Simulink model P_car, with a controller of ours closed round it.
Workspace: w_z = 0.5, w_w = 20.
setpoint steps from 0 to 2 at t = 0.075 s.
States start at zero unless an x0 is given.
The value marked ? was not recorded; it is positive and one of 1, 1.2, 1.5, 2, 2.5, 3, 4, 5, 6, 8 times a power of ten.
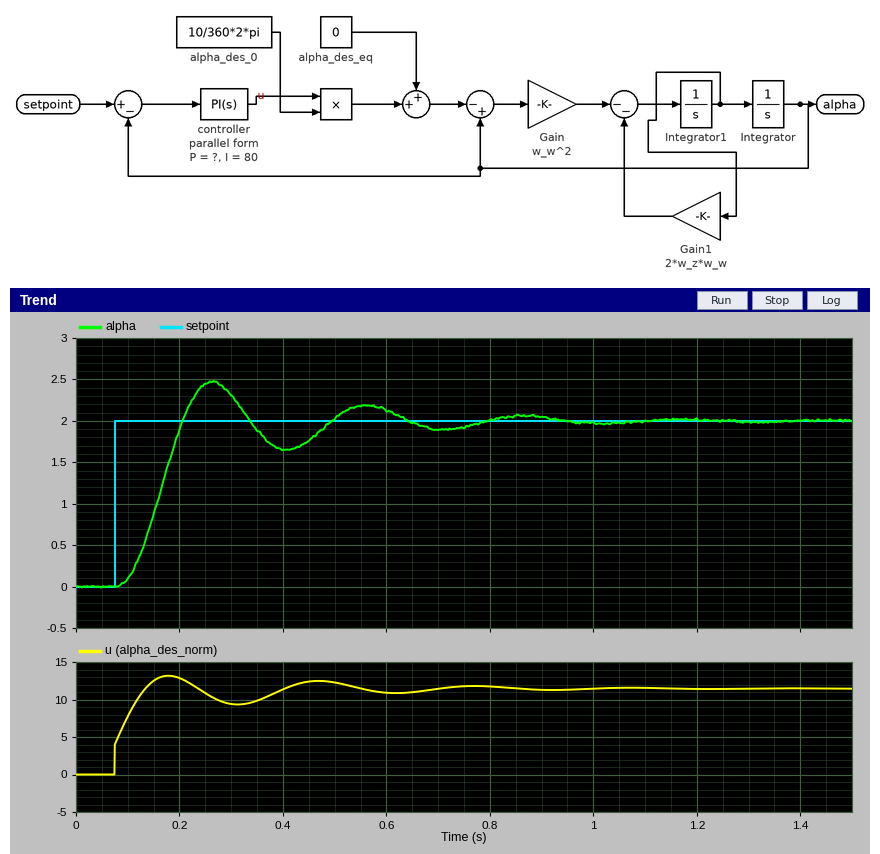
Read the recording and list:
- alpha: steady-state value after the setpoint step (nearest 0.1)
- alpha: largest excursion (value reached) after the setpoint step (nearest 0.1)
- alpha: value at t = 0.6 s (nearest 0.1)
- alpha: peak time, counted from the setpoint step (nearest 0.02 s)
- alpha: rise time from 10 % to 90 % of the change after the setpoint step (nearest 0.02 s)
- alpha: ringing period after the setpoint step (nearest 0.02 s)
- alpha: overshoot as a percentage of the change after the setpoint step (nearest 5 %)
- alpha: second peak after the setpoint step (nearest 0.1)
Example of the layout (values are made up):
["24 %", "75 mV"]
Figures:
["2.0", "2.5", "2.1", "0.18 s", "0.08 s", "0.30 s", "25 %", "2.2"]
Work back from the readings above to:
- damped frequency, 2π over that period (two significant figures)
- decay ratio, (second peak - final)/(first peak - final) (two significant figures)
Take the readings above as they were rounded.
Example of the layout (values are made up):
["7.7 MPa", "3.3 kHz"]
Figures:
["21 rad/s", "0.40"]
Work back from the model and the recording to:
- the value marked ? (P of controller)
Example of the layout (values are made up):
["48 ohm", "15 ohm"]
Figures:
["2"]
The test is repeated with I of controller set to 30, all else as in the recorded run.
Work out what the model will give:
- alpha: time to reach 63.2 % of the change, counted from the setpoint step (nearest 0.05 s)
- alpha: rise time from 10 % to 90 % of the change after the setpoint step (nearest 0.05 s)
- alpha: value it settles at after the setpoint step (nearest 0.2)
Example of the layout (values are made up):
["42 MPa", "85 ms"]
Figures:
["0.15 s", "0.40 s", "2.0"]
